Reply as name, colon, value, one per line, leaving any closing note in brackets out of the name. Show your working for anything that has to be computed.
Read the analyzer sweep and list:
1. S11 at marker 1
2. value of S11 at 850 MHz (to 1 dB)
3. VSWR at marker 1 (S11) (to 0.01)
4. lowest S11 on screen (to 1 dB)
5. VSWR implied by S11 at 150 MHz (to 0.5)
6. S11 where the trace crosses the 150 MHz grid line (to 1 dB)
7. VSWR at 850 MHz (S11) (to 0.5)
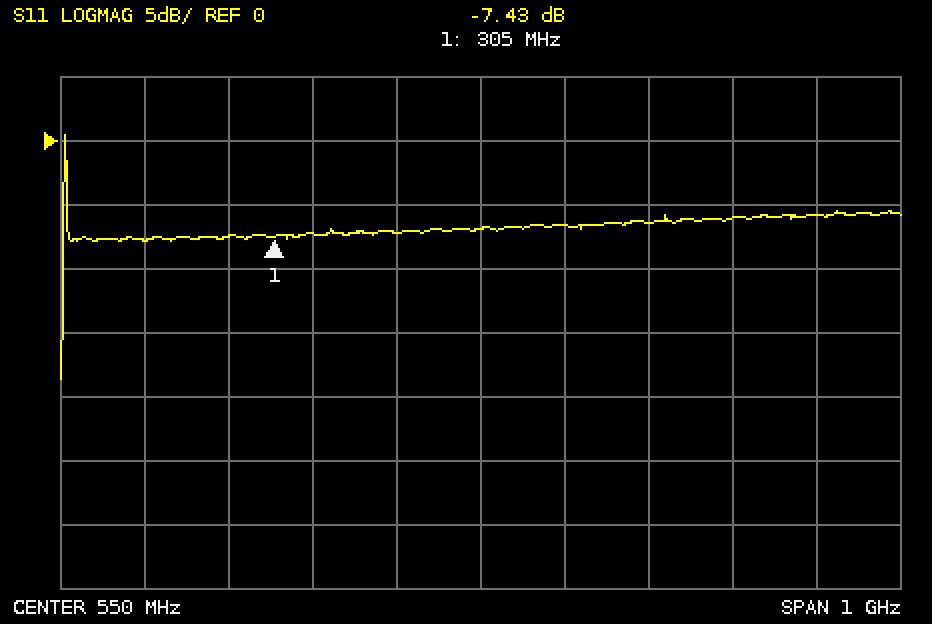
S11 at marker 1: -7.43 dB
value of S11 at 850 MHz: -6 dB
VSWR at marker 1 (S11): (1 + 0.4251)/(1 − 0.4251) ≈ 2.48
lowest S11 on screen: -19 dB
VSWR implied by S11 at 150 MHz: |Γ| = 10^(-8/20) = 0.3981; VSWR = (1 + 0.3981)/(1 − 0.3981) ≈ 2.32, so 2.5 to the nearest 0.5
S11 where the trace crosses the 150 MHz grid line: -8 dB
VSWR at 850 MHz (S11): |Γ| = 10^(-6/20) = 0.5012; VSWR = (1 + 0.5012)/(1 − 0.5012) ≈ 3.0
